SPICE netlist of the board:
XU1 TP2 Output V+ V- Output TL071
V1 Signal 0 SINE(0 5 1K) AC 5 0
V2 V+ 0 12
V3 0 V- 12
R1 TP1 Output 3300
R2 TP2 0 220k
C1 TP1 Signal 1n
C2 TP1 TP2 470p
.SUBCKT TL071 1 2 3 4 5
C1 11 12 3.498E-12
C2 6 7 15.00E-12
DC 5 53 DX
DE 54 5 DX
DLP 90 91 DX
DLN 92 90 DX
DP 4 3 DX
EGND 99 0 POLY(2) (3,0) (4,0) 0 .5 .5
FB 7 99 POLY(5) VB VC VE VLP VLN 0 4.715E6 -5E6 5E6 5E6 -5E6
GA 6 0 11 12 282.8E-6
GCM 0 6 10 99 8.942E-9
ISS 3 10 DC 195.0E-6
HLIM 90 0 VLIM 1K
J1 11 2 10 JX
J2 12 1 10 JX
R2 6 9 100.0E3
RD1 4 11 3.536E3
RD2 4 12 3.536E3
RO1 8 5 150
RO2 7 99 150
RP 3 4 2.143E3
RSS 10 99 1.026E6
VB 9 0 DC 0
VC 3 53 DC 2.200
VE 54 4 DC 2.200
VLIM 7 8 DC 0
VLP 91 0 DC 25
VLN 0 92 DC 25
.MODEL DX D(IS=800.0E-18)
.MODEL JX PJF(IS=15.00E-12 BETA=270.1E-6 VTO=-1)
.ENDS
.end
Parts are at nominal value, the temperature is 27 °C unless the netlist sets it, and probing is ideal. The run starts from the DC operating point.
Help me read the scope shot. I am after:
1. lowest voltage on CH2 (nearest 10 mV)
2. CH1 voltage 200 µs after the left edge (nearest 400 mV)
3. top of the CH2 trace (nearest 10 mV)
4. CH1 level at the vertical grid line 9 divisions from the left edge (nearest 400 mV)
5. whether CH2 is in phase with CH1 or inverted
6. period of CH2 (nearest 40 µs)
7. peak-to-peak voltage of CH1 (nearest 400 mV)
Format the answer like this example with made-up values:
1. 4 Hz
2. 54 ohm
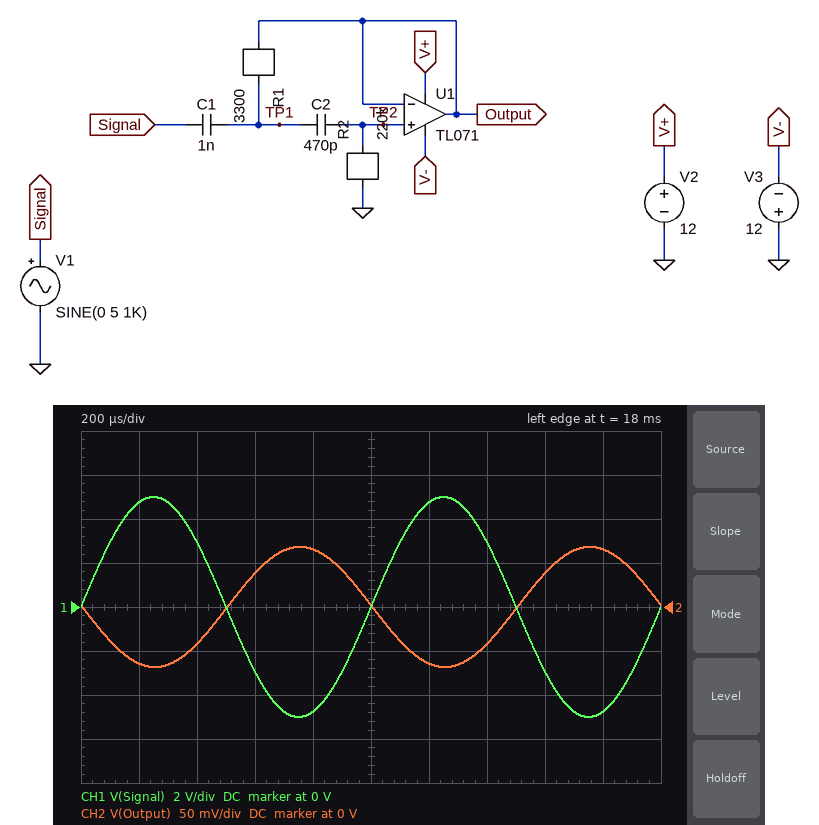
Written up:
1. -70 mV
2. 4.8 V
3. 70 mV
4. -4.8 V
5. inverted
6. 1.00 ms
7. 10.0 V
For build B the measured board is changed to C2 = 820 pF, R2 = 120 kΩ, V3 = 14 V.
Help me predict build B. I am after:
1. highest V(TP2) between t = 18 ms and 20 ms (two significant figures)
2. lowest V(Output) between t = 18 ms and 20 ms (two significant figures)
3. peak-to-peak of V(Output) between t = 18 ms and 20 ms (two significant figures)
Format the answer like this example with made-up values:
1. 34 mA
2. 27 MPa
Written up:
1. 65 mV
2. -65 mV
3. 130 mV
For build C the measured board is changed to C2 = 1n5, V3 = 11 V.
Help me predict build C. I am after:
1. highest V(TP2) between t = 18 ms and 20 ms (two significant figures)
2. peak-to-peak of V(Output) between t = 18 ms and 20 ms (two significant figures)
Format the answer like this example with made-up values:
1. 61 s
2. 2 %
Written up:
1. 220 mV
2. 450 mV
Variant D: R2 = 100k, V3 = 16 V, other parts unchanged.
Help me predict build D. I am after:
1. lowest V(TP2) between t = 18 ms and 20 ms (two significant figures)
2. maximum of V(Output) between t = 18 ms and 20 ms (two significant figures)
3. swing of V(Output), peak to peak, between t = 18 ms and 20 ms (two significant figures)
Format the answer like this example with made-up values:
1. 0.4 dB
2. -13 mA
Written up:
1. -31 mV
2. 31 mV
3. 62 mV
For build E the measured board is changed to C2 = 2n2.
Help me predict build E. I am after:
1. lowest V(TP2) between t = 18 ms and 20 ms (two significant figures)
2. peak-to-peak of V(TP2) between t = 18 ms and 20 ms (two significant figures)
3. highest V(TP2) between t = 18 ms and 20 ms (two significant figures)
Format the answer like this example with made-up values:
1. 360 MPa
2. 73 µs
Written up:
1. -340 mV
2. 670 mV
3. 340 mV
